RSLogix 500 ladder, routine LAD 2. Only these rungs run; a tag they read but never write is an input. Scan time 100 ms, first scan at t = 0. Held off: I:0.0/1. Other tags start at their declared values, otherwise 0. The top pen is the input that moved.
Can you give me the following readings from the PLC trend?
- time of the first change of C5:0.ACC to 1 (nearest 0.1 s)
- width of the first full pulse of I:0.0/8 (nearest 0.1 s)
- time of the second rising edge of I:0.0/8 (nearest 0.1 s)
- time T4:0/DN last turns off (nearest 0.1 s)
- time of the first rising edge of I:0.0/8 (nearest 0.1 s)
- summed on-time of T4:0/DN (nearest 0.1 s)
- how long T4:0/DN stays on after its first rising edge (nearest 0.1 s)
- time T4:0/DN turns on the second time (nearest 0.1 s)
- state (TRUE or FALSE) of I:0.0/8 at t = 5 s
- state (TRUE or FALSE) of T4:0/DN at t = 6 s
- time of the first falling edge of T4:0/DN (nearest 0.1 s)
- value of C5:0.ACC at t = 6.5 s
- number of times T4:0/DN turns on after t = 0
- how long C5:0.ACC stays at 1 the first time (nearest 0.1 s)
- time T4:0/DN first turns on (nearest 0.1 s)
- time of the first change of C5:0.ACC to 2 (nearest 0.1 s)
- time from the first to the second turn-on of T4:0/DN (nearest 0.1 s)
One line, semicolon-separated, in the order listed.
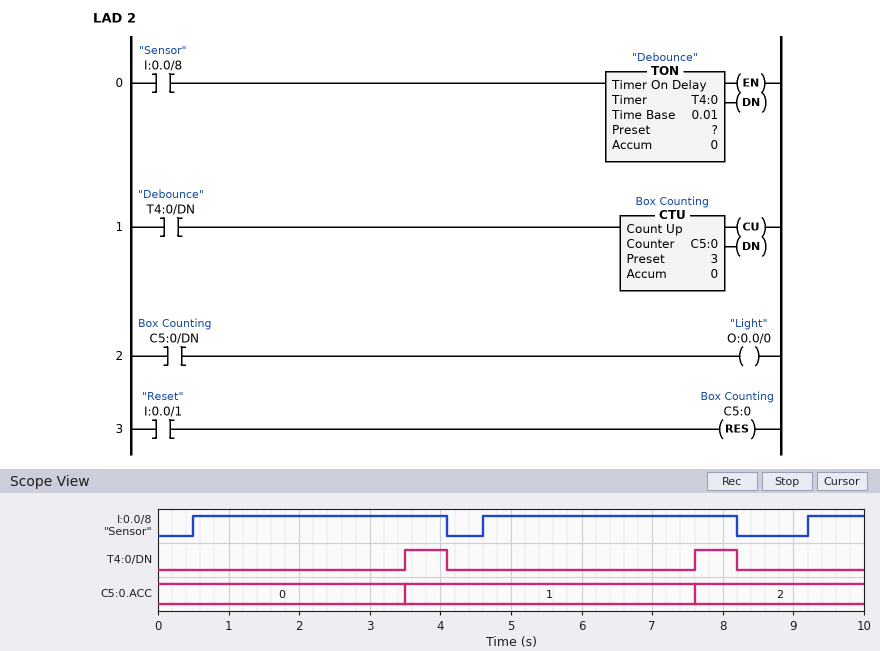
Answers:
3.5 s; 3.6 s; 4.6 s; 8.2 s; 0.5 s; 1.2 s; 0.6 s; 7.6 s; TRUE; FALSE; 4.1 s; 1; 2; 4.1 s; 3.5 s; 7.6 s; 4.1 s
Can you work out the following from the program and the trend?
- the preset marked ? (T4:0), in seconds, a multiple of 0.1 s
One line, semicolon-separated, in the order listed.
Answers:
3.0 s
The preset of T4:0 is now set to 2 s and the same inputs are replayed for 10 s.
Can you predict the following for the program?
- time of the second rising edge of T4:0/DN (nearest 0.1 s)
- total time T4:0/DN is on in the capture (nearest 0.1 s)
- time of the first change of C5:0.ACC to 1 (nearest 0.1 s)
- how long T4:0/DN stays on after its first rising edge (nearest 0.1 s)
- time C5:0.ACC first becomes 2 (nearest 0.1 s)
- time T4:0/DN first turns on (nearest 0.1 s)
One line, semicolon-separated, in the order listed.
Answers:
6.6 s; 3.2 s; 2.5 s; 1.6 s; 6.6 s; 2.5 s
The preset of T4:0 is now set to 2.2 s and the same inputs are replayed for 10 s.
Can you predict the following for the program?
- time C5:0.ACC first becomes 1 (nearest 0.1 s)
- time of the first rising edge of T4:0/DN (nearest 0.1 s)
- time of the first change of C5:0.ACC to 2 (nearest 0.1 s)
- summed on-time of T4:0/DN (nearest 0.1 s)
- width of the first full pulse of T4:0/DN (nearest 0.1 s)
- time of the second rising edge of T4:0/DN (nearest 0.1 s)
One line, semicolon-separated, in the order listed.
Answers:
2.7 s; 2.7 s; 6.8 s; 2.8 s; 1.4 s; 6.8 s
